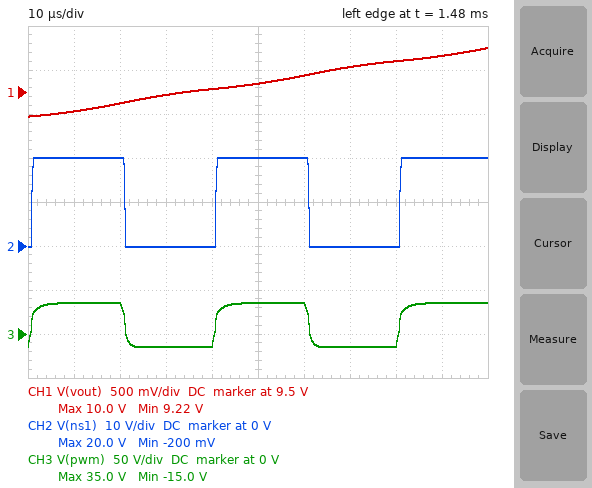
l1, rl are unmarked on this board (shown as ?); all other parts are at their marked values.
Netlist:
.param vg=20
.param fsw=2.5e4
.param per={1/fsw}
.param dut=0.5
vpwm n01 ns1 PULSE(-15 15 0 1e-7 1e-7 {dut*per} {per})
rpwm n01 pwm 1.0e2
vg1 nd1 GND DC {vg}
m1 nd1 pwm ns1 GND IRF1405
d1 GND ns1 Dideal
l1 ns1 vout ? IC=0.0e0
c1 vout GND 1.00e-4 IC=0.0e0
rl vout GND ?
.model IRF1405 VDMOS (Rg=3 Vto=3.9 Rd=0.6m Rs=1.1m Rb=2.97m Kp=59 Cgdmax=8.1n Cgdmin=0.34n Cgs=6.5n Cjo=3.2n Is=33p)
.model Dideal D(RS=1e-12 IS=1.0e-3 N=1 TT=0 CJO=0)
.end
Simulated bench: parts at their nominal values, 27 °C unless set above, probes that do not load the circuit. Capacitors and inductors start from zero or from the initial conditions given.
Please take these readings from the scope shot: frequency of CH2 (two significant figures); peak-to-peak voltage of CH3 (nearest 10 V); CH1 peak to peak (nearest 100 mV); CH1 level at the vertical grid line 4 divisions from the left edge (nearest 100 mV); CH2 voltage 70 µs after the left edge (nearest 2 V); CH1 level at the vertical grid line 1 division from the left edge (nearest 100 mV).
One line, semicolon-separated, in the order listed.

25 kHz; 50 V; 800 mV; 9.5 V; 0 V; 9.3 V
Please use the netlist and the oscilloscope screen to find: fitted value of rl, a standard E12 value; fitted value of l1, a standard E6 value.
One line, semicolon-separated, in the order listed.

6.8 Ω; 330 µH
